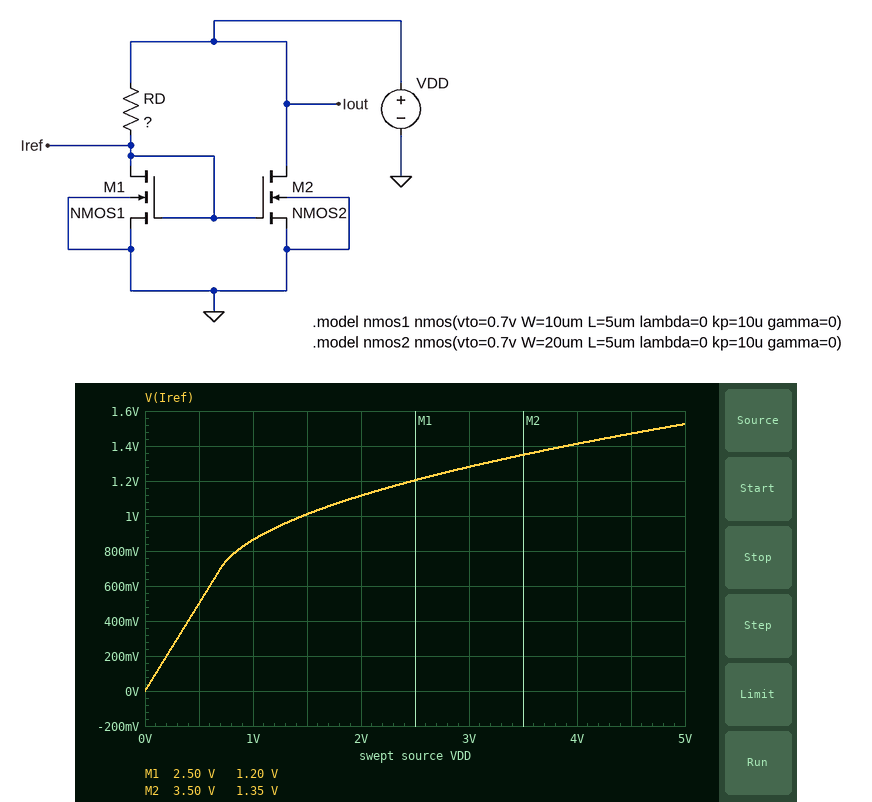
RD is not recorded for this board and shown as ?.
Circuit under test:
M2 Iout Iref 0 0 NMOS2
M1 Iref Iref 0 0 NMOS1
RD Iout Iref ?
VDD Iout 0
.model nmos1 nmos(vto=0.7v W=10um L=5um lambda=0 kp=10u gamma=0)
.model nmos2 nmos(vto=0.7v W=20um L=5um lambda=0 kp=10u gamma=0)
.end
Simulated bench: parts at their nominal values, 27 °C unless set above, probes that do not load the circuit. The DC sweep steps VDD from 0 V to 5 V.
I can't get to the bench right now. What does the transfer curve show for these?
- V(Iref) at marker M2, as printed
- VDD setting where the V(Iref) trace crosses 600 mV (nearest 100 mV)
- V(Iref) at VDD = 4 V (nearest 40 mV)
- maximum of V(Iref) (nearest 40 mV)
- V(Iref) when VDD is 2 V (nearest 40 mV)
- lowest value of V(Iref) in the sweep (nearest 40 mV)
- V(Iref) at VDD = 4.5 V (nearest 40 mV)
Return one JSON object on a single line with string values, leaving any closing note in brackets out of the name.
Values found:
{"V(Iref) at marker M2, as printed": "1.35 V", "VDD setting where the V(Iref) trace crosses 600 mV": "600 mV", "V(Iref) at VDD = 4 V": "1.40 V", "maximum of V(Iref)": "1.52 V", "V(Iref) when VDD is 2 V": "1.12 V", "lowest value of V(Iref) in the sweep": "0 V", "V(Iref) at VDD = 4.5 V": "1.48 V"}
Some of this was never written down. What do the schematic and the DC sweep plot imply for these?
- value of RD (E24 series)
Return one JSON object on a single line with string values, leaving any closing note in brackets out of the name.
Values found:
{"value of RD": "510 kΩ"}
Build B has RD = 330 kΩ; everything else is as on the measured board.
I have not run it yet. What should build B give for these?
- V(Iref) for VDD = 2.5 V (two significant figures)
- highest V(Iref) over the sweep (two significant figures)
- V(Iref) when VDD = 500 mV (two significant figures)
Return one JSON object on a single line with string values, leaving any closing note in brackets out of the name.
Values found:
{"V(Iref) for VDD = 2.5 V": "1.3 V", "highest V(Iref) over the sweep": "1.7 V", "V(Iref) when VDD = 500 mV": "500 mV"}
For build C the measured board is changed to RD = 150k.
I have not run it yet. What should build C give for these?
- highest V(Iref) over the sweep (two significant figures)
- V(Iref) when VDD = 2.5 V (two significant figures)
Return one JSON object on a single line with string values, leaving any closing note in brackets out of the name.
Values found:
{"highest V(Iref) over the sweep": "2.1 V", "V(Iref) when VDD = 2.5 V": "1.5 V"}
